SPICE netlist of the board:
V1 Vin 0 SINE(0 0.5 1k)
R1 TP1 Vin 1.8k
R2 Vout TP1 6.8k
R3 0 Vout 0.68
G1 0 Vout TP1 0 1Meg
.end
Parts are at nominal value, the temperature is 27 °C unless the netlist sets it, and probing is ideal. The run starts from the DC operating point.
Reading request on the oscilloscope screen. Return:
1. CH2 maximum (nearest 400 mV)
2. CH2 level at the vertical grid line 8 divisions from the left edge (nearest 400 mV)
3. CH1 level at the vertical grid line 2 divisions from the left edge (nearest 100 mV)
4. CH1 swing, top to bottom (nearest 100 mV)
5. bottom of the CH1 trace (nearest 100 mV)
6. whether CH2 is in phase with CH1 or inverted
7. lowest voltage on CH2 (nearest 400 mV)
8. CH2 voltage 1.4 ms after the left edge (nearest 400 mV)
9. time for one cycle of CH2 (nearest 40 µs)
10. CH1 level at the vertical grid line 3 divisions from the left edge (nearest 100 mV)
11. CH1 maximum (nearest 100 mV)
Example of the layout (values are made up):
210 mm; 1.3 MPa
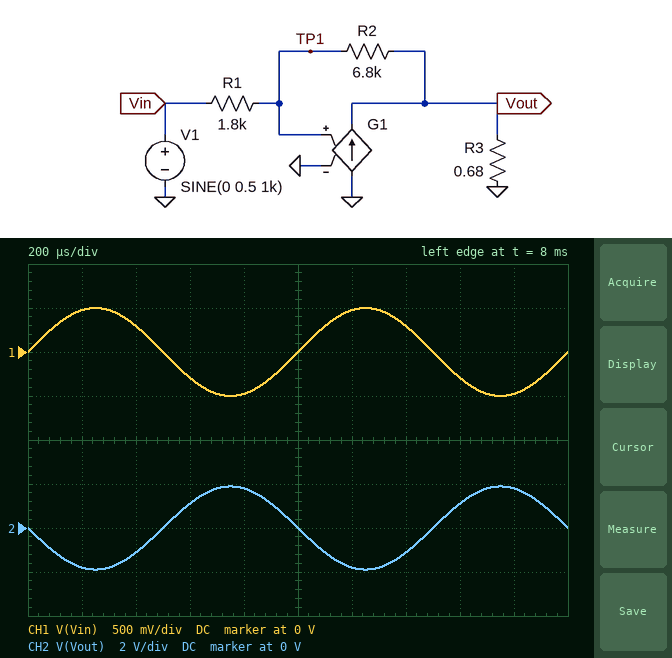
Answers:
2.0 V; 1.2 V; 300 mV; 1.0 V; -500 mV; inverted; -2.0 V; -1.2 V; 1.00 ms; -300 mV; 500 mV
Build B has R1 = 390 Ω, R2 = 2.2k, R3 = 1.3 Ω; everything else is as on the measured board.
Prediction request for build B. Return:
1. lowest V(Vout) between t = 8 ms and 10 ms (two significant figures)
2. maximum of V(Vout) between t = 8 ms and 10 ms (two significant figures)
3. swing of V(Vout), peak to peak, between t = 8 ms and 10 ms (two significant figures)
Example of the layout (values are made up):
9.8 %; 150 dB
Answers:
-2.8 V; 2.8 V; 5.6 V
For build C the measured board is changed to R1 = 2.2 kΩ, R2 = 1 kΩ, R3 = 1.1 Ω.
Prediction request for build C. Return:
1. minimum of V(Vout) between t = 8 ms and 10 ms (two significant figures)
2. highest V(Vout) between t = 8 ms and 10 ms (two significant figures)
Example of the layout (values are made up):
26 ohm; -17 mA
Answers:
-230 mV; 230 mV
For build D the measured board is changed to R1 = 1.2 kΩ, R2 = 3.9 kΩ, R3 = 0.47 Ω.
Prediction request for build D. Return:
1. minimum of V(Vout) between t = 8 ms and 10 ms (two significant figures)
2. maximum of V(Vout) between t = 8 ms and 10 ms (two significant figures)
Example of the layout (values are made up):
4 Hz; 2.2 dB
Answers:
-1.6 V; 1.6 V
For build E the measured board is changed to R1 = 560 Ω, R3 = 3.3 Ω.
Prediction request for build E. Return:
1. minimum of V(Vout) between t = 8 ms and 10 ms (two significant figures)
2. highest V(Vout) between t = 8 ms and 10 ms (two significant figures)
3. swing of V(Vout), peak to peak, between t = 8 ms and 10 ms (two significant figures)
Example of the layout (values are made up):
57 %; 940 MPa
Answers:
-6.1 V; 6.1 V; 12 V
